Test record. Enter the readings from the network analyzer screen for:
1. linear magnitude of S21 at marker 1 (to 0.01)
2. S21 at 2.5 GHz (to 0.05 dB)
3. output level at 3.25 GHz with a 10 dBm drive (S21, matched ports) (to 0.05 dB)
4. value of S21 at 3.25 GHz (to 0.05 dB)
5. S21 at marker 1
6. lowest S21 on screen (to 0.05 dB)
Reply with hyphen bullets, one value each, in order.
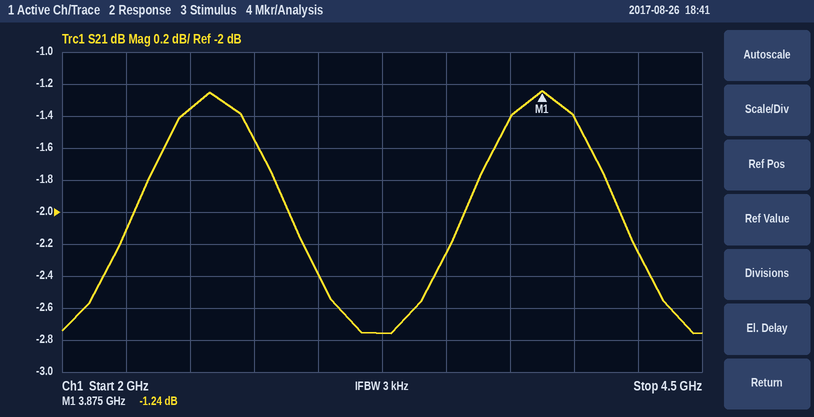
- 0.87
- -1.35 dB
- 7.25 dBm
- -2.75 dB
- -1.24 dB
- -2.75 dB
